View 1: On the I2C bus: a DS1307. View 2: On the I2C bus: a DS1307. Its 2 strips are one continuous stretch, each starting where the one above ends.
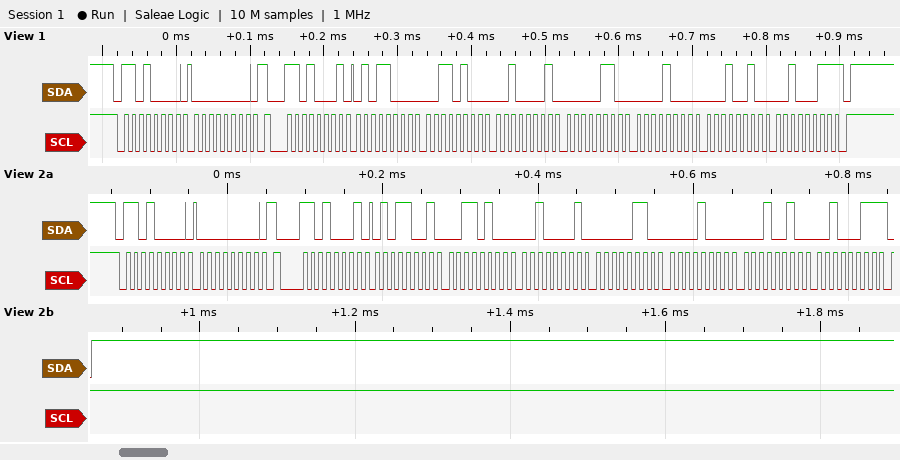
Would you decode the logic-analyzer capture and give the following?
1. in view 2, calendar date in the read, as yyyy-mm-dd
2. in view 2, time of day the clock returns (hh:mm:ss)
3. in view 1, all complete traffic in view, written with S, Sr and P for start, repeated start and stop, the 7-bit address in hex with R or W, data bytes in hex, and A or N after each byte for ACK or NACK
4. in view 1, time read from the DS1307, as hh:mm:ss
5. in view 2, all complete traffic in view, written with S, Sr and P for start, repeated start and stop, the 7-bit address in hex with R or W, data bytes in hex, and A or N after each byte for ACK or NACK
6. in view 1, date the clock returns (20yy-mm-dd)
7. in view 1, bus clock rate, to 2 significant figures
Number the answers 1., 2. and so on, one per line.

1. 2023-12-08
2. 21:34:59
3. S 68W A 00 A Sr 68R A 58 A 34 A 21 A 06 A 08 A 12 A 23 N P
4. 21:34:58
5. S 68W A 00 A Sr 68R A 59 A 34 A 21 A 06 A 08 A 12 A 23 N P
6. 2023-12-08
7. 100 kHz
